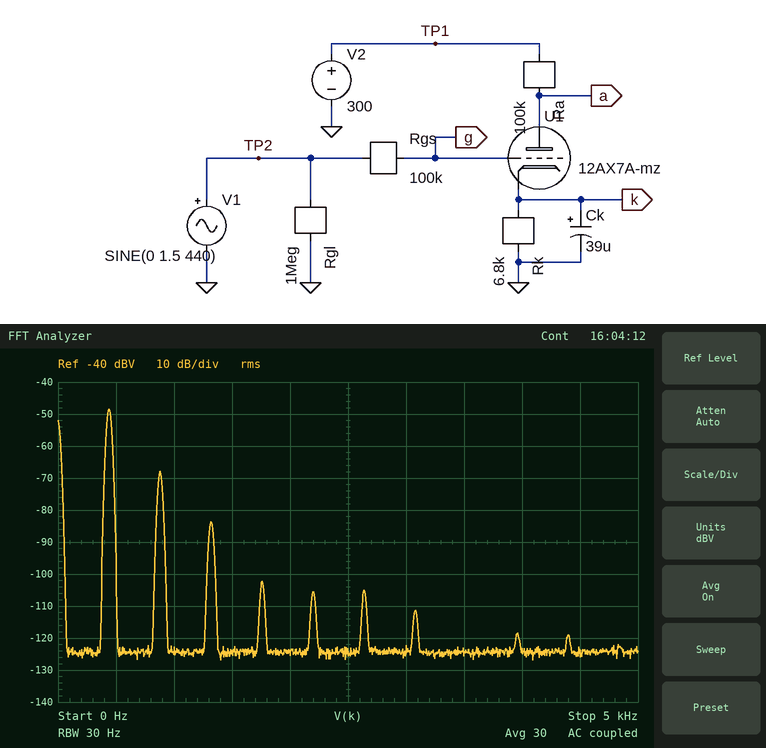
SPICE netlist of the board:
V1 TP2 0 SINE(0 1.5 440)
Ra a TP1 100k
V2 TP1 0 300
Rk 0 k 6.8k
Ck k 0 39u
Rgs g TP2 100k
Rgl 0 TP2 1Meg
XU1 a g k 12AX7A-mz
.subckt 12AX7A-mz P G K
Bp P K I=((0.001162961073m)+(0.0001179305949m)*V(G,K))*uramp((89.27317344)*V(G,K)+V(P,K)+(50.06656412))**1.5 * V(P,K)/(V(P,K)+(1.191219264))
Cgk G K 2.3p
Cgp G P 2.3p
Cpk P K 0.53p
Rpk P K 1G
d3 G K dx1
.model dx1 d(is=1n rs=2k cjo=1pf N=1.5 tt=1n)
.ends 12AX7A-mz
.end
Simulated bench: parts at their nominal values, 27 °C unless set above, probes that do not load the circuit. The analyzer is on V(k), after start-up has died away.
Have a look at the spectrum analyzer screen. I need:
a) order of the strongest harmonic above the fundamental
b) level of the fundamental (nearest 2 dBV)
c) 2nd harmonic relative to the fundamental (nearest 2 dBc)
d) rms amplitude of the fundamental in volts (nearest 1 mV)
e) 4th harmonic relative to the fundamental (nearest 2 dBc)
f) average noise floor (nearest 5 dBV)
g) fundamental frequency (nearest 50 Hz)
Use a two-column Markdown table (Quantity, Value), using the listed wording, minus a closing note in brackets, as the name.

| Quantity | Value |
|---|---|
| order of the strongest harmonic above the fundamental | 2 |
| level of the fundamental | -48 dBV |
| 2nd harmonic relative to the fundamental | -20 dBc |
| rms amplitude of the fundamental in volts | 4 mV |
| 4th harmonic relative to the fundamental | -54 dBc |
| average noise floor | -125 dBV |
| fundamental frequency | 450 Hz |
